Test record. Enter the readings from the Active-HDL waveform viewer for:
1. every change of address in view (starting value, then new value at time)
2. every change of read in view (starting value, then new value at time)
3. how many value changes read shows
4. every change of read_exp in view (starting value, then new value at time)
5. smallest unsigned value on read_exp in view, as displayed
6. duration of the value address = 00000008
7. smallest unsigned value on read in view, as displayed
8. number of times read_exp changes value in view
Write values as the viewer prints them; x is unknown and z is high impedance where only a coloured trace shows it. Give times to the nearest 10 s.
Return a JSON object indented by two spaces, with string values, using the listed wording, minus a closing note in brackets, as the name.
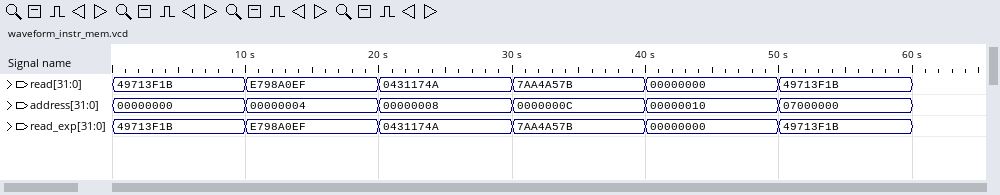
{
  "every change of address in view": "00000000, 00000004 at 10 s, 00000008 at 20 s, 0000000C at 30 s, 00000010 at 40 s, 07000000 at 50 s",
  "every change of read in view": "49713F1B, E798A0EF at 10 s, 0431174A at 20 s, 7AA4A57B at 30 s, 00000000 at 40 s, 49713F1B at 50 s",
  "how many value changes read shows": "5",
  "every change of read_exp in view": "49713F1B, E798A0EF at 10 s, 0431174A at 20 s, 7AA4A57B at 30 s, 00000000 at 40 s, 49713F1B at 50 s",
  "smallest unsigned value on read_exp in view, as displayed": "00000000",
  "duration of the value address = 00000008": "10 s",
  "smallest unsigned value on read in view, as displayed": "00000000",
  "number of times read_exp changes value in view": "5"
}
